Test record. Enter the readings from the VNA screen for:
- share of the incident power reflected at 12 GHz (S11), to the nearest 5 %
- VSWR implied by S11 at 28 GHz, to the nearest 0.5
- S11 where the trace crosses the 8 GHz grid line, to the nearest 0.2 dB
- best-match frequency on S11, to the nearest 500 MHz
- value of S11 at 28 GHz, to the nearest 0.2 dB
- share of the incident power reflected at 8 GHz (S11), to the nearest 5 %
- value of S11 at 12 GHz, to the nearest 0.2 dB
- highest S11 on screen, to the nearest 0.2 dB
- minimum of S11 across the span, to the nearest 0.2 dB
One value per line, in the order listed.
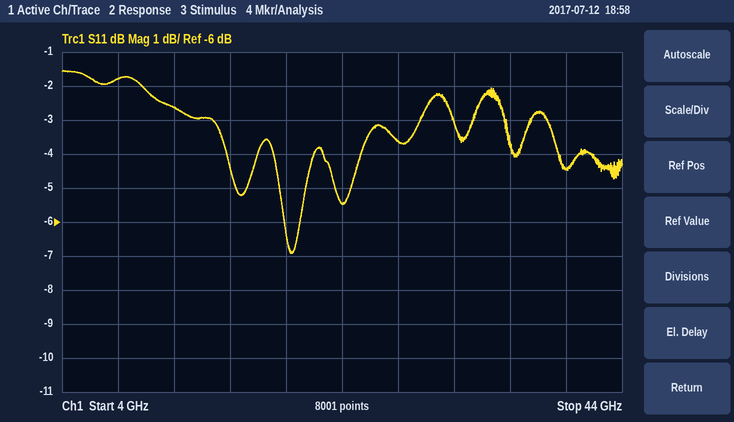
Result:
55 %
5.0
-1.8 dB
20.5 GHz
-3.6 dB
65 %
-2.6 dB
-1.6 dB
-7.0 dB
